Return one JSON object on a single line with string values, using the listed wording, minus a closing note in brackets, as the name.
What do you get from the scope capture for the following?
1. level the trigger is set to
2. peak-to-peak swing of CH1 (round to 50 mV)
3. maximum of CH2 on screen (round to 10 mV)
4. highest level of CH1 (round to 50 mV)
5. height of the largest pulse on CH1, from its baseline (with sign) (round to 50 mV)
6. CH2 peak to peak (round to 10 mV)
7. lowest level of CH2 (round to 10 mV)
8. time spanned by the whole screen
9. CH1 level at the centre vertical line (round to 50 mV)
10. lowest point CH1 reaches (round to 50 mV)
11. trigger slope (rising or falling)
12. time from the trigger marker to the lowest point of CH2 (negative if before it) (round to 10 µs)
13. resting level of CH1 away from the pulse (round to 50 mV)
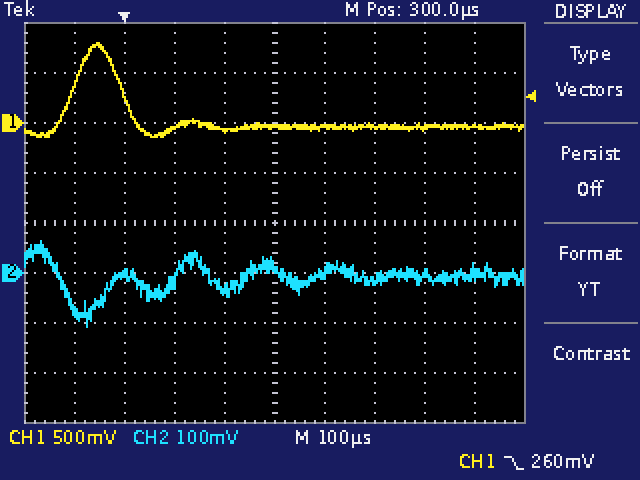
{"level the trigger is set to": "260 mV", "peak-to-peak swing of CH1": "950 mV", "maximum of CH2 on screen": "60 mV", "highest level of CH1": "800 mV", "height of the largest pulse on CH1, from its baseline (with sign)": "+850 mV", "CH2 peak to peak": "170 mV", "lowest level of CH2": "-110 mV", "time spanned by the whole screen": "1 ms", "CH1 level at the centre vertical line": "-50 mV", "lowest point CH1 reaches": "-150 mV", "trigger slope": "falling", "time from the trigger marker to the lowest point of CH2 (negative if before it)": "-70 µs", "resting level of CH1 away from the pulse": "-50 mV"}
